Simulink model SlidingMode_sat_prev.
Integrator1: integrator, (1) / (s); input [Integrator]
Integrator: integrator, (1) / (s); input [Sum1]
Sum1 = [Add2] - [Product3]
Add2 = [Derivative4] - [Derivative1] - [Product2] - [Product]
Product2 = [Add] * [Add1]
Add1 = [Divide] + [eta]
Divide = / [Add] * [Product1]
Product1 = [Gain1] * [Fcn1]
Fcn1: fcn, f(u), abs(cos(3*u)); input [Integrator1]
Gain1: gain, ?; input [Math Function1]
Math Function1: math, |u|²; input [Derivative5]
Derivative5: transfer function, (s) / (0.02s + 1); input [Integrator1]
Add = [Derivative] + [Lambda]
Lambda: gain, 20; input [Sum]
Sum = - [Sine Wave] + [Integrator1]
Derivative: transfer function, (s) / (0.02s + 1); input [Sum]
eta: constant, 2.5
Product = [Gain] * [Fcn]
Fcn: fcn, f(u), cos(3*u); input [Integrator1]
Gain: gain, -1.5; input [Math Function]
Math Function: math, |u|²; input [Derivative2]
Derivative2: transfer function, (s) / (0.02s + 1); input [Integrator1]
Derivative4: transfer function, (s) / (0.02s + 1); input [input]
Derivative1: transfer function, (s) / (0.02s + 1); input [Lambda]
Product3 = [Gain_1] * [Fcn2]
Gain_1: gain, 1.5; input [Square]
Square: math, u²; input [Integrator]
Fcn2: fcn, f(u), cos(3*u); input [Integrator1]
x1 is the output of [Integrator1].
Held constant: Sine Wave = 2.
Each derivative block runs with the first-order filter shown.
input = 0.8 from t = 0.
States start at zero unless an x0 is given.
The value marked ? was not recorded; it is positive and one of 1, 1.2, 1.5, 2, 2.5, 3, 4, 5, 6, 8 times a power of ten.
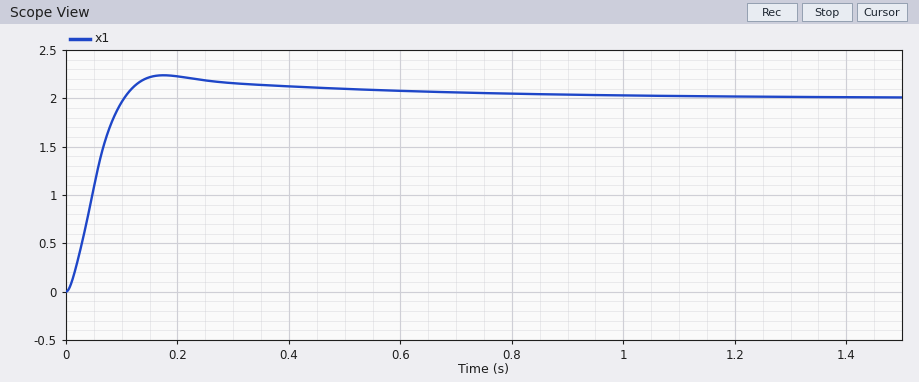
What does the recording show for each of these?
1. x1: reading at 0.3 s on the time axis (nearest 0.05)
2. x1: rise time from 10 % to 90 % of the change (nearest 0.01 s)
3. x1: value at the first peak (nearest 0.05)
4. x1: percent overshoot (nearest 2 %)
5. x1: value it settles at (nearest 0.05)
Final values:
2.15
0.07 s
2.25
12 %
2.00
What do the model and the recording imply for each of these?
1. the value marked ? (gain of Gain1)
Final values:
0.4
